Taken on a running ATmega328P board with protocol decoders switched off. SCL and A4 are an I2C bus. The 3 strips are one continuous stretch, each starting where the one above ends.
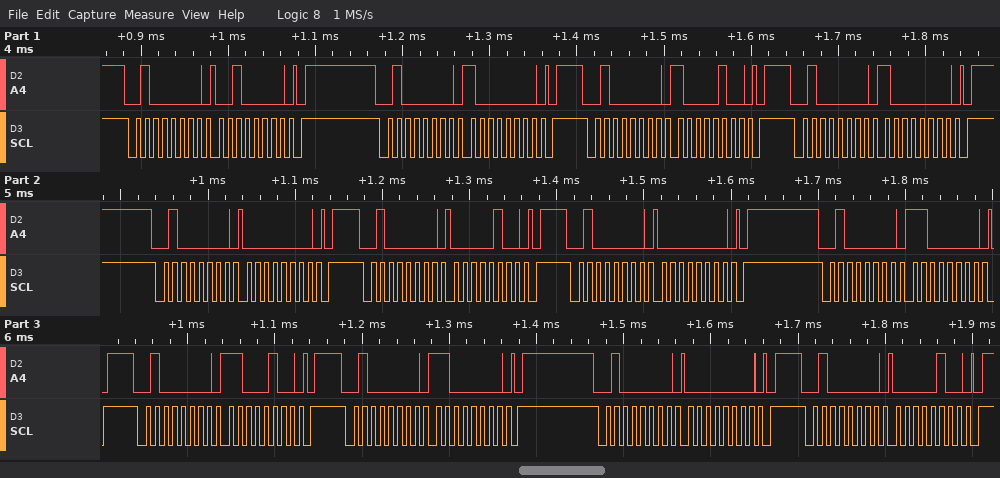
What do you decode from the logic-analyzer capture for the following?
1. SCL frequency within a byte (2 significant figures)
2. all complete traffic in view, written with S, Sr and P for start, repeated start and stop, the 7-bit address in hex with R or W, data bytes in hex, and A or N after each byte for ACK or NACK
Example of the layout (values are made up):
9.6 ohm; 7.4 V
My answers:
100 kHz; S 20W A 20 A P S 20W A 80 A P S 20W A 84 A P S 20W A 80 A P S 20W A 00 A P S 20W A 04 A P S 20W A 00 A P S 20W A C0 A P S 20W A C4 A P S 20W A C0 A P S 20W A 00 A P S 20W A 04 A P
